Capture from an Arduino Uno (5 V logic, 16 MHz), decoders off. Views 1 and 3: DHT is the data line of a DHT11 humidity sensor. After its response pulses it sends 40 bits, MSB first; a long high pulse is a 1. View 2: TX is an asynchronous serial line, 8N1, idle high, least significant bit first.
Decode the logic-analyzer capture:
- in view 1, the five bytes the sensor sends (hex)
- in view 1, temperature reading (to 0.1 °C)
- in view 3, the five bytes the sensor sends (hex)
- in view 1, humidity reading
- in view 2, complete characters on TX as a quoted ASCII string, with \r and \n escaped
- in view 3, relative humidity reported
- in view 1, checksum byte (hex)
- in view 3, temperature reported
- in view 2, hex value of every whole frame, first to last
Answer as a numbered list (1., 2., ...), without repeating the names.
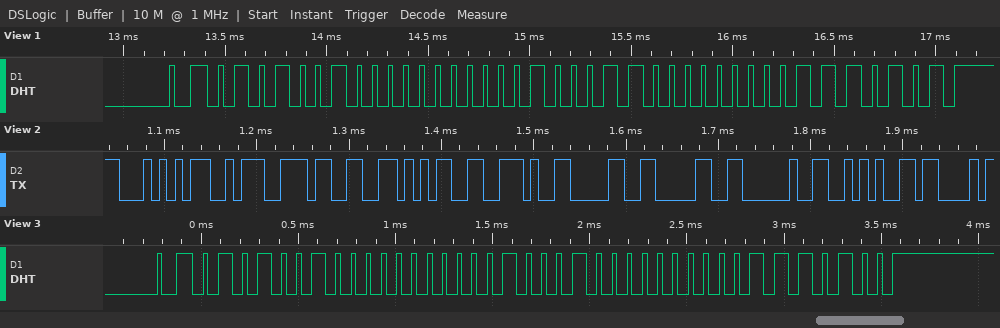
1. 52 00 23 00 75
2. 35.0 °C
3. 52 00 22 00 74
4. 82 %
5. "T:35.00 *C"
6. 82 %
7. 0x75
8. 34.0 °C
9. 54 3A 33 35 2E 30 30 20 2A 43
